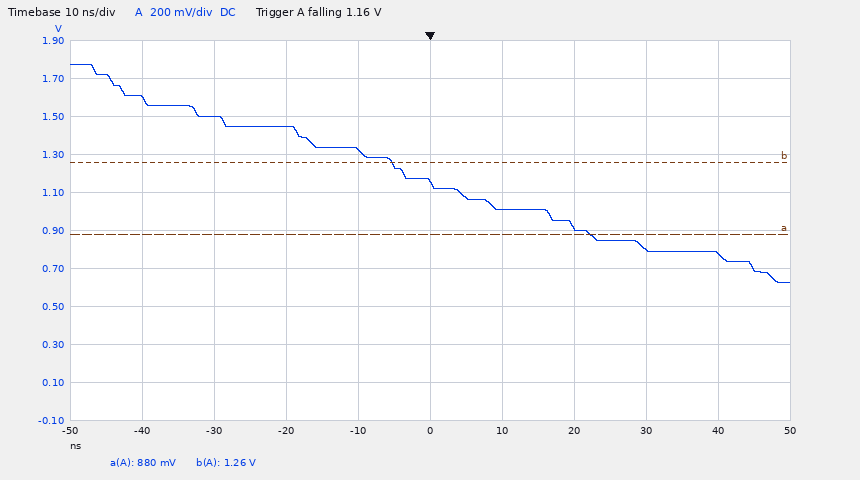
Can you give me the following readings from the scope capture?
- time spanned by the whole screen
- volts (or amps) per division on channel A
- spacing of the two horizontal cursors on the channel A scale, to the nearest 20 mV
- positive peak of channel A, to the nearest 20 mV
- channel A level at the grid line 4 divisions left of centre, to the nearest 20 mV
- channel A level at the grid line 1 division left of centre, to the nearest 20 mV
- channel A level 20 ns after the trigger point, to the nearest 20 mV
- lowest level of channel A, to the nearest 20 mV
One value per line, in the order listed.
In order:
100 ns
200 mV
380 mV
1.78 V
1.60 V
1.32 V
920 mV
620 mV
